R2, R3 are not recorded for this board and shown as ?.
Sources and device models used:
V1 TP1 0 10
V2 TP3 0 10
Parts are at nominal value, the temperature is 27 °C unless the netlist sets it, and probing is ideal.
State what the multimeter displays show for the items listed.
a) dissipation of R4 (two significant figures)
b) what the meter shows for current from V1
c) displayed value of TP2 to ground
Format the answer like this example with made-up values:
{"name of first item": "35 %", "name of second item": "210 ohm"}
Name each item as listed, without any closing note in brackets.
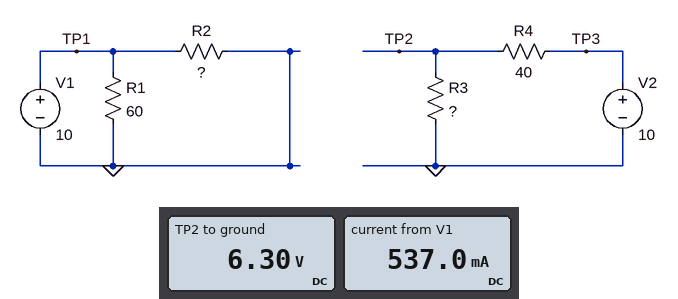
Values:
{"dissipation of R4": "340 mW", "what the meter shows for current from V1": "537.0 mA", "displayed value of TP2 to ground": "6.30 V"}
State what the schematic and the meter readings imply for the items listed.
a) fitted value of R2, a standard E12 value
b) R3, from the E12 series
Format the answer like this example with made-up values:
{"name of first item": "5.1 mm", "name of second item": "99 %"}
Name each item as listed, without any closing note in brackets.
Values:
{"fitted value of R2, a standard E12 value": "27 Ω", "R3, from the E12 series": "68 Ω"}
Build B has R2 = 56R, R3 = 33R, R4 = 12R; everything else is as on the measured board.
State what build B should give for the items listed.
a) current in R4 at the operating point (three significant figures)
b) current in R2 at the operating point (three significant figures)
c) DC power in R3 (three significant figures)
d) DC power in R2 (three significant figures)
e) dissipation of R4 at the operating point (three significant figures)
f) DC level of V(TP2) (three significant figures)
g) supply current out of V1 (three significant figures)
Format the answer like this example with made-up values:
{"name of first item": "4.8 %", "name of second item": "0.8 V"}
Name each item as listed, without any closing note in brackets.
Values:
{"current in R4 at the operating point": "222 mA", "current in R2 at the operating point": "179 mA", "DC power in R3": "1.63 W", "DC power in R2": "1.79 W", "dissipation of R4 at the operating point": "593 mW", "DC level of V(TP2)": "7.33 V", "supply current out of V1": "345 mA"}
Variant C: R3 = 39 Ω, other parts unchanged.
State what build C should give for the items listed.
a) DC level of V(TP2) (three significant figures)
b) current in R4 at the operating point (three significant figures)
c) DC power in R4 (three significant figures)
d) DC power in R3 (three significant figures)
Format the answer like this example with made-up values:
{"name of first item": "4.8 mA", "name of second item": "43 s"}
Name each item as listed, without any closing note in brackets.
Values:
{"DC level of V(TP2)": "4.94 V", "current in R4 at the operating point": "127 mA", "DC power in R4": "641 mW", "DC power in R3": "625 mW"}
